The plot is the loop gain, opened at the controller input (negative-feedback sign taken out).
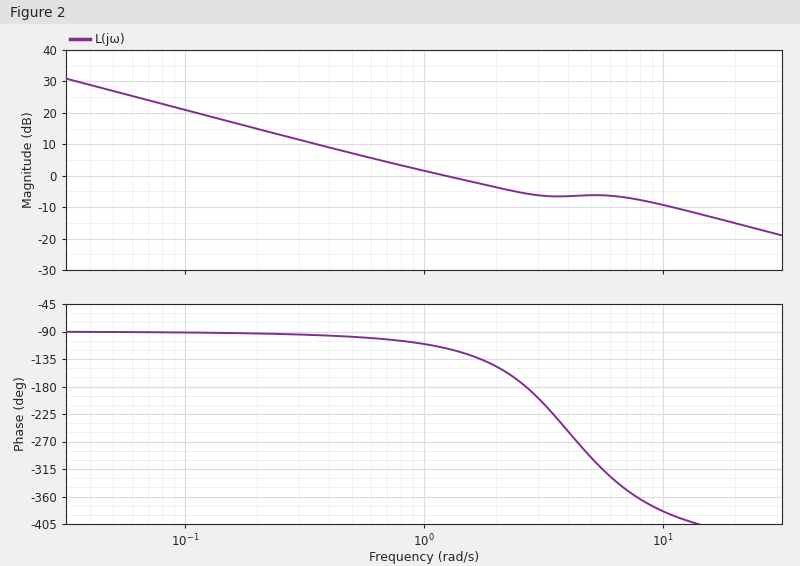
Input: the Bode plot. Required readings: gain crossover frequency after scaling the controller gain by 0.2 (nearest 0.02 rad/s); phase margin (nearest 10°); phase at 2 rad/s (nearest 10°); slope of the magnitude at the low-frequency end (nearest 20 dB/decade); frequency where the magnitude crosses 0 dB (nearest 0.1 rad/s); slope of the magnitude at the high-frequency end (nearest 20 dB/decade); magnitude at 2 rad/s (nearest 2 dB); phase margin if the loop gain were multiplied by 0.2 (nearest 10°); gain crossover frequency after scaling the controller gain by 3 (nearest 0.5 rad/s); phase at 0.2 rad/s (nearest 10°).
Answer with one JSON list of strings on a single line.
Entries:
["0.22 rad/s", "60°", "-150°", "-20 dB/decade", "1.2 rad/s", "-20 dB/decade", "-4 dB", "90°", "10.5 rad/s", "-90°"]
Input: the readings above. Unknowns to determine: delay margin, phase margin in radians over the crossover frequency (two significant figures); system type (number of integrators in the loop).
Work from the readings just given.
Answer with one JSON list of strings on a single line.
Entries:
["0.87 s", "1"]
